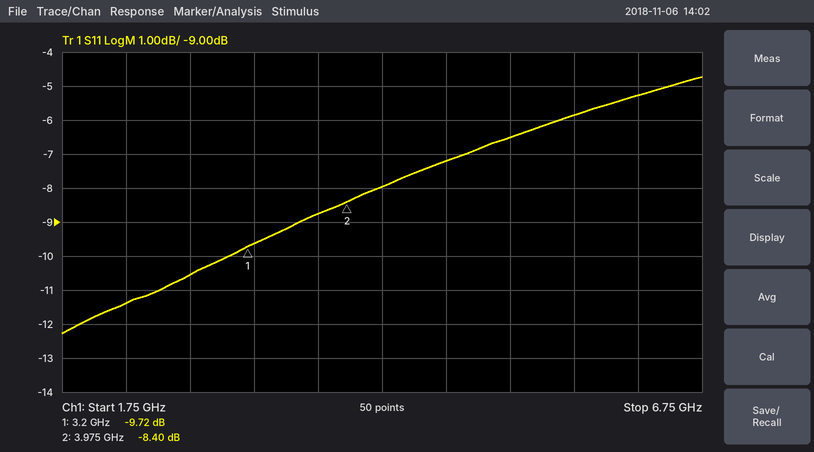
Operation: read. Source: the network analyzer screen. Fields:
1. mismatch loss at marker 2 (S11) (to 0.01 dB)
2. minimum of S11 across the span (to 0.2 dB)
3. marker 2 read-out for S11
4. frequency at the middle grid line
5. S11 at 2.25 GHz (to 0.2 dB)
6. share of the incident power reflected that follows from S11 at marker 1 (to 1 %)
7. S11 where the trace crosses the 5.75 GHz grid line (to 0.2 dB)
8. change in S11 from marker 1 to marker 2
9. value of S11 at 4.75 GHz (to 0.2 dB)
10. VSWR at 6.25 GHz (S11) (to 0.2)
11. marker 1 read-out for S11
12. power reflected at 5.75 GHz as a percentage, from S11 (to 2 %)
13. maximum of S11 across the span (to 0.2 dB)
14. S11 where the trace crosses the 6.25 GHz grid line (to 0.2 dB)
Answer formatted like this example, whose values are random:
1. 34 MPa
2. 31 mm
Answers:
1. 0.68 dB
2. -12.2 dB
3. -8.40 dB
4. 4.25 GHz
5. -11.4 dB
6. 11 %
7. -5.8 dB
8. 1.32 dB
9. -7.2 dB
10. 3.4
11. -9.72 dB
12. 26 %
13. -4.8 dB
14. -5.2 dB
